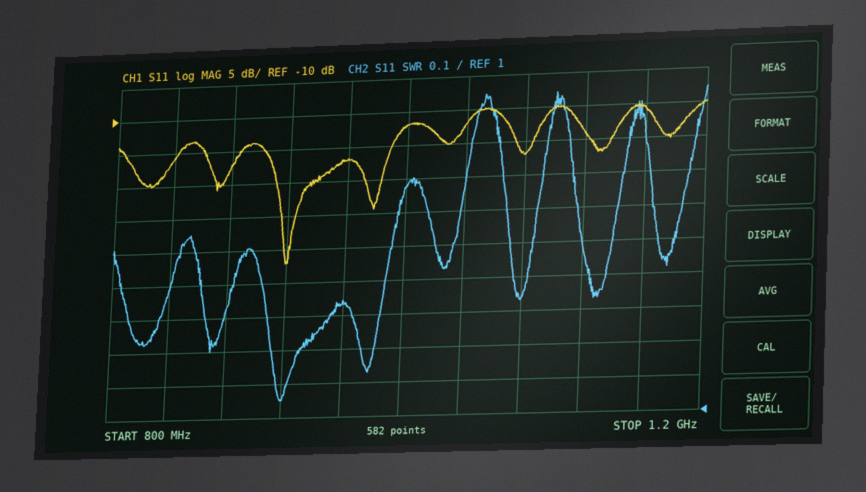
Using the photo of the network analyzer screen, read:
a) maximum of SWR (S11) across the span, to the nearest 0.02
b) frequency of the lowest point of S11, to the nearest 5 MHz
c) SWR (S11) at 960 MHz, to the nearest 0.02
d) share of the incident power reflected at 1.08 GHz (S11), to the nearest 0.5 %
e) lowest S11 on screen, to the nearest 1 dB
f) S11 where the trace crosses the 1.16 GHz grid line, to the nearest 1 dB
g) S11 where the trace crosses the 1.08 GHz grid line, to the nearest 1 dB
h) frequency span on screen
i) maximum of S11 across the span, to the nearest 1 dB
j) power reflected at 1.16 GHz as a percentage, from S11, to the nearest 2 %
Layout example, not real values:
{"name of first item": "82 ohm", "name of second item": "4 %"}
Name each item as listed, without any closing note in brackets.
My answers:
{"maximum of SWR (S11) across the span, to the nearest 0.02": "1.94", "frequency of the lowest point of S11, to the nearest 5 MHz": "920 MHz", "SWR (S11) at 960 MHz, to the nearest 0.02": "1.34", "share of the incident power reflected at 1.08 GHz (S11), to the nearest 0.5 %": "2.0 %", "lowest S11 on screen, to the nearest 1 dB": "-32 dB", "S11 where the trace crosses the 1.16 GHz grid line, to the nearest 1 dB": "-11 dB", "S11 where the trace crosses the 1.08 GHz grid line, to the nearest 1 dB": "-17 dB", "frequency span on screen": "400 MHz", "maximum of S11 across the span, to the nearest 1 dB": "-10 dB", "power reflected at 1.16 GHz as a percentage, from S11, to the nearest 2 %": "8 %"}
